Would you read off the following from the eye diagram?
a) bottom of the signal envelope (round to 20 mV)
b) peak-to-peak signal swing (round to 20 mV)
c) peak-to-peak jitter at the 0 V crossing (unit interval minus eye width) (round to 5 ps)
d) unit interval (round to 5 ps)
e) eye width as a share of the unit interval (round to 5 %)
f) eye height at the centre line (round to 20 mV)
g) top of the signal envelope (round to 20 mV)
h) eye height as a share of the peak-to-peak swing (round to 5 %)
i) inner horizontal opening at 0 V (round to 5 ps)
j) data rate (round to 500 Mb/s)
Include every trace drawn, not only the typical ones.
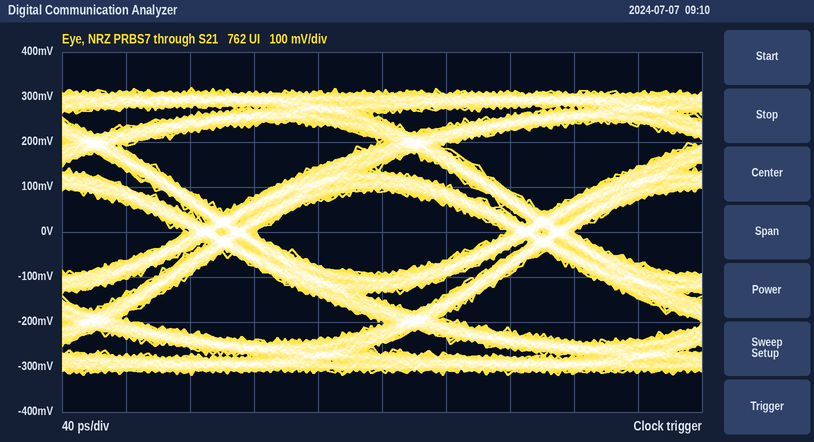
-320 mV
640 mV
45 ps
200 ps
80 %
180 mV
320 mV
30 %
155 ps
5.0 Gb/s
